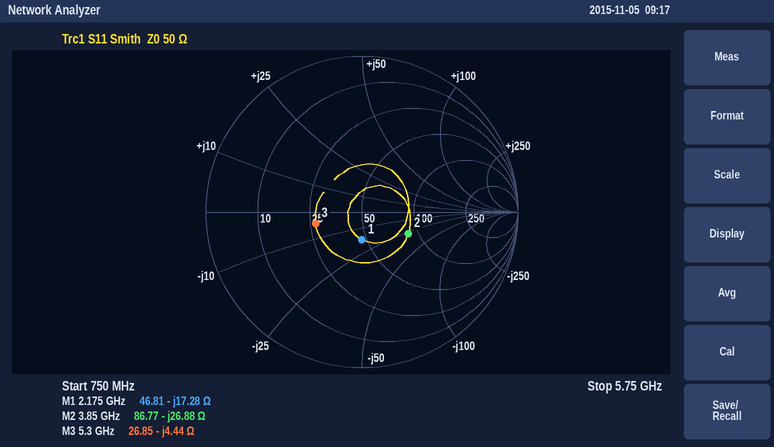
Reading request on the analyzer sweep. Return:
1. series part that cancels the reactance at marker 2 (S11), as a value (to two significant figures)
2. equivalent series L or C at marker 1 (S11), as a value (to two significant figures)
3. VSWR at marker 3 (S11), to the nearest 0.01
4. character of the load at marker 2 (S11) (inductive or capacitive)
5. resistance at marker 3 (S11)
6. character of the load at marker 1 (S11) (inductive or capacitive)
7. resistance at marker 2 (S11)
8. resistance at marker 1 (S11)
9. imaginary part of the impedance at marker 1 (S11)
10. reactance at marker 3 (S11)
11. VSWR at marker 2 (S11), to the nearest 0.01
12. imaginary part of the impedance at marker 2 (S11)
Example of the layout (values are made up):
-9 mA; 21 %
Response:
1.1 nH; 4.2 pF; 1.88; capacitive; 26.85 Ω; capacitive; 86.77 Ω; 46.81 Ω; -17.28 Ω; -4.44 Ω; 1.97; -26.88 Ω
